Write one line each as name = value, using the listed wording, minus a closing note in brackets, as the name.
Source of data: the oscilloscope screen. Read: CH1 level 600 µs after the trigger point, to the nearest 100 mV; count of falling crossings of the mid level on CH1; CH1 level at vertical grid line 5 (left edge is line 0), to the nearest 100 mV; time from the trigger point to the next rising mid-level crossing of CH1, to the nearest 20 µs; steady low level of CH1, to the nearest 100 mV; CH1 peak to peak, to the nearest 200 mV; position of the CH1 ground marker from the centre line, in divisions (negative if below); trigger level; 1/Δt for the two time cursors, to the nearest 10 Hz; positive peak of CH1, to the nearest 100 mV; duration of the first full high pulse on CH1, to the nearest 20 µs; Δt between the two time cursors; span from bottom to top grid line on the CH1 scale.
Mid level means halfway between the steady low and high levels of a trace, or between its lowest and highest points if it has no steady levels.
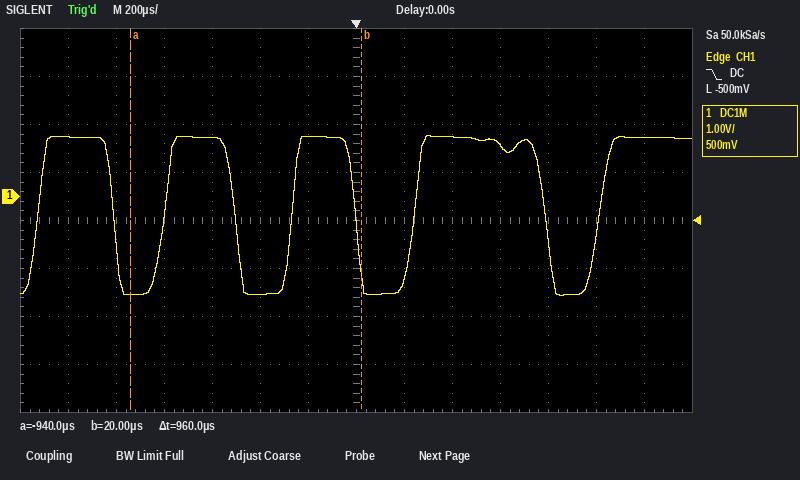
CH1 level 600 µs after the trigger point, to the nearest 100 mV = 1.1 V
count of falling crossings of the mid level on CH1 = 4
CH1 level at vertical grid line 5 (left edge is line 0), to the nearest 100 mV = -2.0 V
time from the trigger point to the next rising mid-level crossing of CH1, to the nearest 20 µs = 240 µs
steady low level of CH1, to the nearest 100 mV = -2.0 V
CH1 peak to peak, to the nearest 200 mV = 3.4 V
position of the CH1 ground marker from the centre line, in divisions = +0.5 div
trigger level = -500 mV
1/Δt for the two time cursors, to the nearest 10 Hz = 1.04 kHz
positive peak of CH1, to the nearest 100 mV = 1.3 V
duration of the first full high pulse on CH1, to the nearest 20 µs = 320 µs
Δt between the two time cursors = 960 µs
span from bottom to top grid line on the CH1 scale = 8 V
